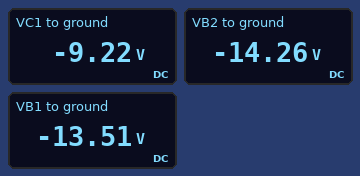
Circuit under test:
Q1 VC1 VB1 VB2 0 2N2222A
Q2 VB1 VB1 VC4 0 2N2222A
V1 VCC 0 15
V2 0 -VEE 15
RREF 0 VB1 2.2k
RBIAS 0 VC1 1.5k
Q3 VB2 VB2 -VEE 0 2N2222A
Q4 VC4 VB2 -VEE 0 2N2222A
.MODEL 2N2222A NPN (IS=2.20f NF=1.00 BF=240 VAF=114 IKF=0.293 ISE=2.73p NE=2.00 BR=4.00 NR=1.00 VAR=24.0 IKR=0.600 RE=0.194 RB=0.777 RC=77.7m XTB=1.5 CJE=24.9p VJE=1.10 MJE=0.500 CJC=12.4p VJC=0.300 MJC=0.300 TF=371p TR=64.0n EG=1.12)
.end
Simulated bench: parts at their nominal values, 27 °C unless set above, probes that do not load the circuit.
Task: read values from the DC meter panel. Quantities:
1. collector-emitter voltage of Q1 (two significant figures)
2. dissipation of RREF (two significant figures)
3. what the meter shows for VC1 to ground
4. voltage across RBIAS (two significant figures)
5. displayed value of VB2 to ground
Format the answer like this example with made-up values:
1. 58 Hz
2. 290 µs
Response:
1. 5.0 V
2. 83 mW
3. -9.22 V
4. 9.2 V
5. -14.26 V
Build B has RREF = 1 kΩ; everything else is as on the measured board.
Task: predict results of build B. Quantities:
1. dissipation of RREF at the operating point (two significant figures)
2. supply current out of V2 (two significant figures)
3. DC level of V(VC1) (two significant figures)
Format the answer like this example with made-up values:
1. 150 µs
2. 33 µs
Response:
1. 180 mW
2. 23 mA
3. -14 V
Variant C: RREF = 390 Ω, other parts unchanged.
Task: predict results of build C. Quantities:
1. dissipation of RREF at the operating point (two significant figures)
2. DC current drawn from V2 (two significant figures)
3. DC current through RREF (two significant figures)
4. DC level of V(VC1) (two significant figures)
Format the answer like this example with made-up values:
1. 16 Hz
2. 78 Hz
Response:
1. 460 mW
2. 44 mA
3. 34 mA
4. -14 V
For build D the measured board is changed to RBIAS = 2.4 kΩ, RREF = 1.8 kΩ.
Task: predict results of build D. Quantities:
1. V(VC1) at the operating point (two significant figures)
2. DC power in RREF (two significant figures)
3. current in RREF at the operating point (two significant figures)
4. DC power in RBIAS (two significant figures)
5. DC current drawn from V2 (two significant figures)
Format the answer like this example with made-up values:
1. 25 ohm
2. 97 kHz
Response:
1. -14 V
2. 100 mW
3. 7.5 mA
4. 84 mW
5. 13 mA
